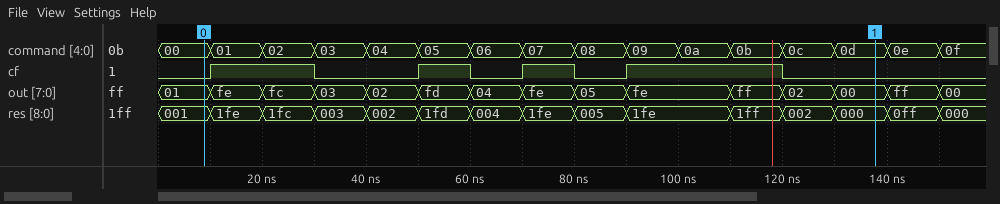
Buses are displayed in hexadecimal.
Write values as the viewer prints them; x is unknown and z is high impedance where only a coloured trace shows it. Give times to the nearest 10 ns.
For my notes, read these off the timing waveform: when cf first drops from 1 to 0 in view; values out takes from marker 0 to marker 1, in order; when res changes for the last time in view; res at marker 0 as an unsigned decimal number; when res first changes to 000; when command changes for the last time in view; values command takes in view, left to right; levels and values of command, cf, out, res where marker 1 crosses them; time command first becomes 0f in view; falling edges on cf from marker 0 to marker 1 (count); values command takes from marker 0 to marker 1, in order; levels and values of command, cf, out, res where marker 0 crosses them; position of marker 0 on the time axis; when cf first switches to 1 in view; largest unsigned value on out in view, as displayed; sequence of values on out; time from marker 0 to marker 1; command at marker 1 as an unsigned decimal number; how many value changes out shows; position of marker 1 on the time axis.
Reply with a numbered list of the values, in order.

1. 30 ns
2. 01, fe, fc, 03, 02, fd, 04, fe, 05, fe, ff, 02, 00
3. 150 ns
4. 1
5. 130 ns
6. 150 ns
7. 00, 01, 02, 03, 04, 05, 06, 07, 08, 09, 0a, 0b, 0c, 0d, 0e, 0f
8. command=0d, cf=0, out=00, res=000
9. 150 ns
10. 4
11. 00, 01, 02, 03, 04, 05, 06, 07, 08, 09, 0a, 0b, 0c, 0d
12. command=00, cf=0, out=01, res=001
13. 10 ns
14. 10 ns
15. ff
16. 01, fe, fc, 03, 02, fd, 04, fe, 05, fe, ff, 02, 00, ff, 00
17. 130 ns
18. 13
19. 14
20. 140 ns
